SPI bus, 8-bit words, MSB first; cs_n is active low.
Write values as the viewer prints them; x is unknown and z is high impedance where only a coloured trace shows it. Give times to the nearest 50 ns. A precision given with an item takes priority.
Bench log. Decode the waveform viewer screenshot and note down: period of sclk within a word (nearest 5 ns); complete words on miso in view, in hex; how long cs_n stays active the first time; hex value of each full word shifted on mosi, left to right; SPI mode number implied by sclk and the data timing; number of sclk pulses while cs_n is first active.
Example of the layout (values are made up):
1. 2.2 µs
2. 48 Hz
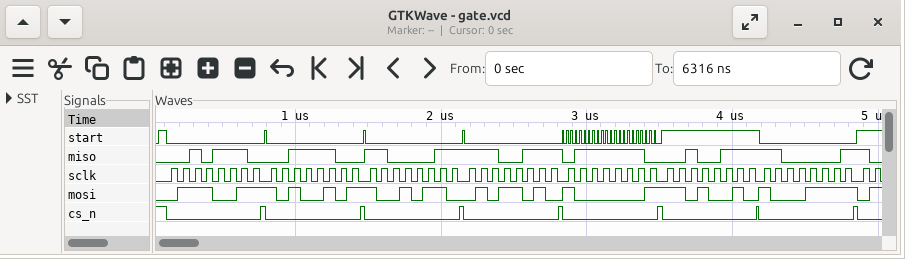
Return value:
1. 80 ns
2. 2E, 3C, C3, E7, 7E, 27, C1
3. 650 ns
4. 73, A5, 96, 5A, 81, D2, 8F
5. 0
6. 8
